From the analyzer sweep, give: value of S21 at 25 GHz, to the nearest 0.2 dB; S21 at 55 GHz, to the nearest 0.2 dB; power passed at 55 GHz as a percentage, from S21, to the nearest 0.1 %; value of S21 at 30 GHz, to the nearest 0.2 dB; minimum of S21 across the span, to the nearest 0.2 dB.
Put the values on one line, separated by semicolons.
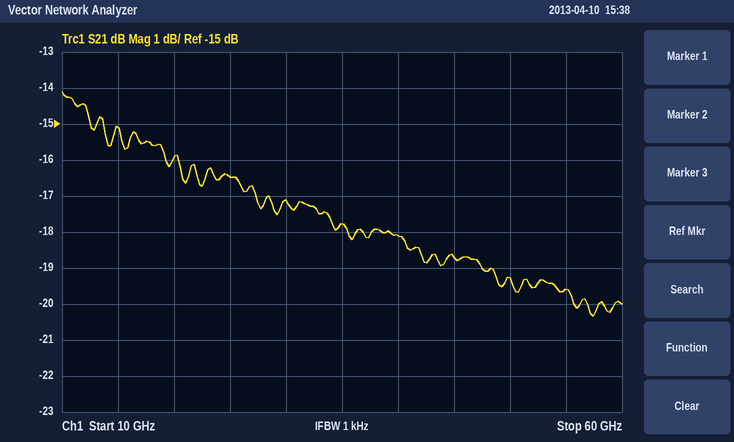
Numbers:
-16.4 dB; -19.6 dB; 1.1 %; -17.2 dB; -20.4 dB
